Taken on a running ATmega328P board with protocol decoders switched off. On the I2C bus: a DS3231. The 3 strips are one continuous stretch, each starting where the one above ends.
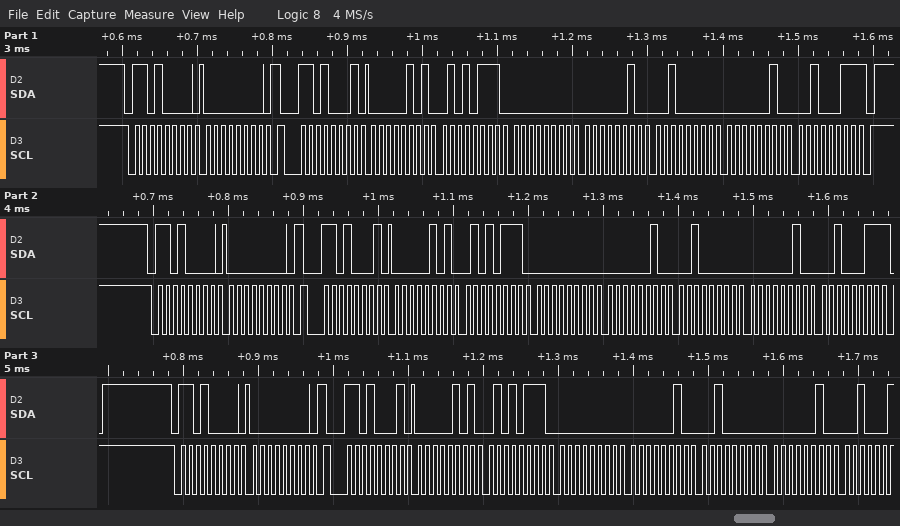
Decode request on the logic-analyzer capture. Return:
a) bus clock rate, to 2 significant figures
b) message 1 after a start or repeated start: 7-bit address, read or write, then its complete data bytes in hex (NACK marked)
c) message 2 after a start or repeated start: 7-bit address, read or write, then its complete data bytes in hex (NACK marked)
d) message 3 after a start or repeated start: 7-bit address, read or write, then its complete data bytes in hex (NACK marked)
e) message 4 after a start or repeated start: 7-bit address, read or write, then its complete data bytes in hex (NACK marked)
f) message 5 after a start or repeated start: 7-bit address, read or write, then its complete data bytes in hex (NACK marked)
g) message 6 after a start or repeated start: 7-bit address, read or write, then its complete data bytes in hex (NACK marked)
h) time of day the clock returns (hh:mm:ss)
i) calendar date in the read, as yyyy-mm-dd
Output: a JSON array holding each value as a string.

["100 kHz", "0x68 write: 00", "0x68 read: 05 57 00 02 20 02 23 NACK", "0x68 write: 00", "0x68 read: 05 57 00 02 20 02 23 NACK", "0x68 write: 00", "0x68 read: 05 57 00 02 20 02", "00:57:05", "2023-02-20"]
